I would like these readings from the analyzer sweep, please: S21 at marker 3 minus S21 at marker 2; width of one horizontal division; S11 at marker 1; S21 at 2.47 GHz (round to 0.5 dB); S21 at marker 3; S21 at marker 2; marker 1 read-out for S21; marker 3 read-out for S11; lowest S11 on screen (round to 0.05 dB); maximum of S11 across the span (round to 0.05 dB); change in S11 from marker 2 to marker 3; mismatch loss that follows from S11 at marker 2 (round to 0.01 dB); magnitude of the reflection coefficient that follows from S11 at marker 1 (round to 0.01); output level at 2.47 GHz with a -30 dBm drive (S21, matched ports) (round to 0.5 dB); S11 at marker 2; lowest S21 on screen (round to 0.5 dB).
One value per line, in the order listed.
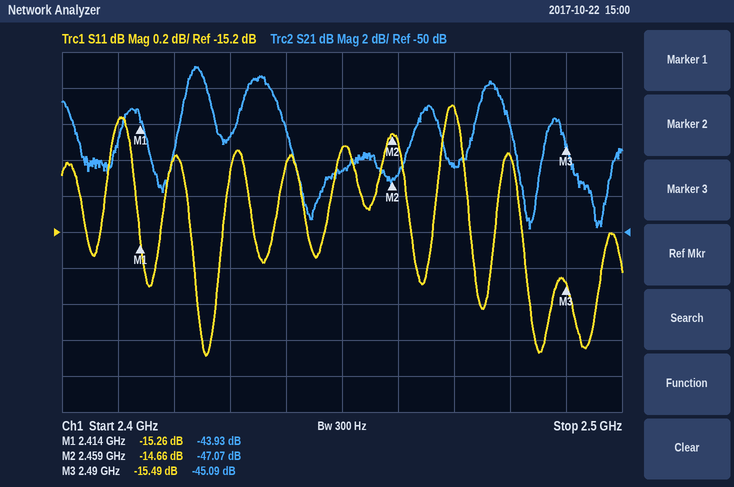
1.98 dB
10 MHz
-15.26 dB
-46.5 dB
-45.09 dB
-47.07 dB
-43.93 dB
-15.49 dB
-15.90 dB
-14.50 dB
-0.83 dB
0.15 dB
0.17
-76.5 dBm
-14.66 dB
-50.0 dB
